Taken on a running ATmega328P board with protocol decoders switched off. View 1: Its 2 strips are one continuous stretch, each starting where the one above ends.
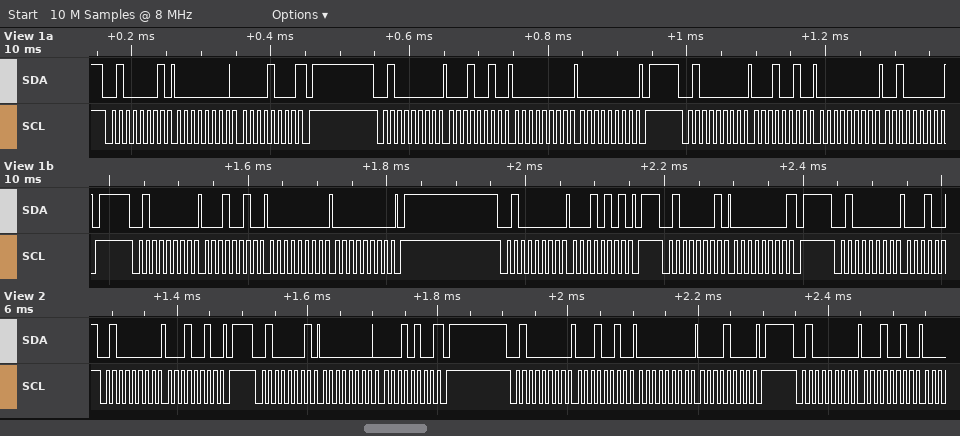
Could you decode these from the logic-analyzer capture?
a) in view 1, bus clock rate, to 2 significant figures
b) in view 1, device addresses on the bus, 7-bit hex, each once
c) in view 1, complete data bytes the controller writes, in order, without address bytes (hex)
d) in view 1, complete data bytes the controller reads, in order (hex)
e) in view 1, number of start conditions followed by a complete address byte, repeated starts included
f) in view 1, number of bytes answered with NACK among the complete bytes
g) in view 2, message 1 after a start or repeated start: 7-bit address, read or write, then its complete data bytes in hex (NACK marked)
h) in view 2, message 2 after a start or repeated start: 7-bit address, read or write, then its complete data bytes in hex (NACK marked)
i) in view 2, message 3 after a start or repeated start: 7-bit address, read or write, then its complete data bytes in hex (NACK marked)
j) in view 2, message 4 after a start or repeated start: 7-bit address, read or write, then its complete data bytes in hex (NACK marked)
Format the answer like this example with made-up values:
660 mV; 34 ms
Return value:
100 kHz; 0x20; 12 00 00 12 00 20 12 00 00 15; 00 08 00; 7; 2; 0x20 write: 12; 0x20 read: 00 14 NACK; 0x20 write: 12 00 08; 0x20 write: 12
